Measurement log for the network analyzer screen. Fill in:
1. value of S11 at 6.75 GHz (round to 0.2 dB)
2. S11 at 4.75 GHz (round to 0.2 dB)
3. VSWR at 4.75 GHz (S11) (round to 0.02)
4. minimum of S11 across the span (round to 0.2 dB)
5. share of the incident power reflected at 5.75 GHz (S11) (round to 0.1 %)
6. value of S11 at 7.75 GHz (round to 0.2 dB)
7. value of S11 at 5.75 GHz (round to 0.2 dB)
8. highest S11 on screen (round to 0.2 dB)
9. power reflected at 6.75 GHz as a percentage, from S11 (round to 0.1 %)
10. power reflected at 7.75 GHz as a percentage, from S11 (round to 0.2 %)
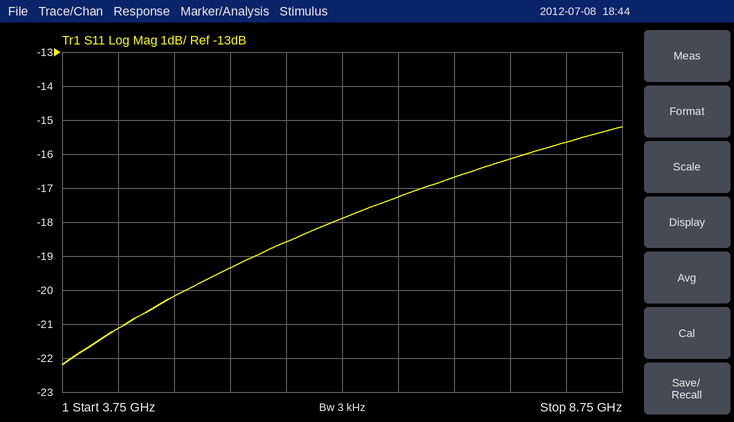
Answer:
-17.2 dB
-20.2 dB
1.22
-22.2 dB
1.4 %
-16.2 dB
-18.6 dB
-15.2 dB
1.9 %
2.4 %
